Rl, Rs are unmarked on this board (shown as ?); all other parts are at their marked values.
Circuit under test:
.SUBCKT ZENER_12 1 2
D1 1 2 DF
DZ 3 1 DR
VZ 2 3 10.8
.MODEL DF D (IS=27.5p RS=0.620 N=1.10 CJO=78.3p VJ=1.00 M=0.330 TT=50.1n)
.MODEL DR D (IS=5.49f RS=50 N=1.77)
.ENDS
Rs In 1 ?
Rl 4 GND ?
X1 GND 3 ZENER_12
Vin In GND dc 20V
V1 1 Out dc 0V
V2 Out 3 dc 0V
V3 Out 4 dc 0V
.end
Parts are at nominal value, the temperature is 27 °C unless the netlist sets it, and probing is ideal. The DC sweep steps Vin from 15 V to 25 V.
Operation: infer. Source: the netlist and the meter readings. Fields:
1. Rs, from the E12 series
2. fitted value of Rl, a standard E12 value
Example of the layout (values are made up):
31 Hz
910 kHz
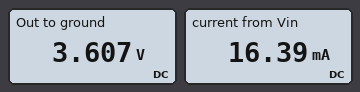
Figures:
1 kΩ
220 Ω
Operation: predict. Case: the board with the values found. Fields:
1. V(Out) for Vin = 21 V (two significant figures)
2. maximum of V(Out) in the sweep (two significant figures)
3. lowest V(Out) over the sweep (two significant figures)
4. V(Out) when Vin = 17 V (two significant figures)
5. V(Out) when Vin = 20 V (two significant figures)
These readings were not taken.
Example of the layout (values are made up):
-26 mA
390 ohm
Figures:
3.8 V
4.5 V
2.7 V
3.1 V
3.6 V
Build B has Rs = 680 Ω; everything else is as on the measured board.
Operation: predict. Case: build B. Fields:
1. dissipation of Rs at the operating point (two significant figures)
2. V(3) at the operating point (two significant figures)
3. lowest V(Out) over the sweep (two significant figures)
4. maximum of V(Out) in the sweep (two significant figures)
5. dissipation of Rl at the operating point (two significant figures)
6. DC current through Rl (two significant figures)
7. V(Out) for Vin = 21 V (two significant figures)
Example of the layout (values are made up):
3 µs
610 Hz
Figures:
340 mW
4.9 V
3.7 V
6.1 V
110 mW
22 mA
5.1 V
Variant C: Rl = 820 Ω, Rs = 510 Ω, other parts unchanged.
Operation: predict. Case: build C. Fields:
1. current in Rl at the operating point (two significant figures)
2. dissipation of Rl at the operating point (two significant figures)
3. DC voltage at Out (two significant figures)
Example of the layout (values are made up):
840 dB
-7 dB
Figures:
15 mA
180 mW
12 V
